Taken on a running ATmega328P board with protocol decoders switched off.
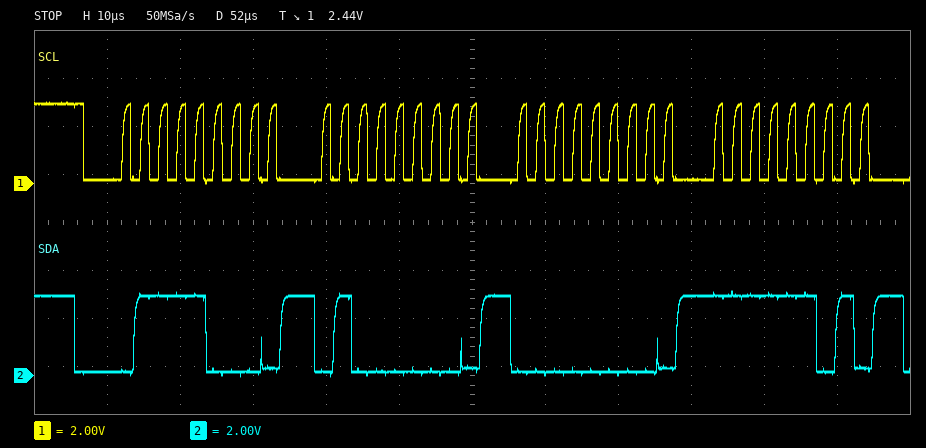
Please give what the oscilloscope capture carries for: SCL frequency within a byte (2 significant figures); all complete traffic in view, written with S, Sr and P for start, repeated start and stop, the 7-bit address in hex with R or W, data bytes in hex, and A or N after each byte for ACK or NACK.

400 kHz
S 3CW A 40 A 00 A FD A
